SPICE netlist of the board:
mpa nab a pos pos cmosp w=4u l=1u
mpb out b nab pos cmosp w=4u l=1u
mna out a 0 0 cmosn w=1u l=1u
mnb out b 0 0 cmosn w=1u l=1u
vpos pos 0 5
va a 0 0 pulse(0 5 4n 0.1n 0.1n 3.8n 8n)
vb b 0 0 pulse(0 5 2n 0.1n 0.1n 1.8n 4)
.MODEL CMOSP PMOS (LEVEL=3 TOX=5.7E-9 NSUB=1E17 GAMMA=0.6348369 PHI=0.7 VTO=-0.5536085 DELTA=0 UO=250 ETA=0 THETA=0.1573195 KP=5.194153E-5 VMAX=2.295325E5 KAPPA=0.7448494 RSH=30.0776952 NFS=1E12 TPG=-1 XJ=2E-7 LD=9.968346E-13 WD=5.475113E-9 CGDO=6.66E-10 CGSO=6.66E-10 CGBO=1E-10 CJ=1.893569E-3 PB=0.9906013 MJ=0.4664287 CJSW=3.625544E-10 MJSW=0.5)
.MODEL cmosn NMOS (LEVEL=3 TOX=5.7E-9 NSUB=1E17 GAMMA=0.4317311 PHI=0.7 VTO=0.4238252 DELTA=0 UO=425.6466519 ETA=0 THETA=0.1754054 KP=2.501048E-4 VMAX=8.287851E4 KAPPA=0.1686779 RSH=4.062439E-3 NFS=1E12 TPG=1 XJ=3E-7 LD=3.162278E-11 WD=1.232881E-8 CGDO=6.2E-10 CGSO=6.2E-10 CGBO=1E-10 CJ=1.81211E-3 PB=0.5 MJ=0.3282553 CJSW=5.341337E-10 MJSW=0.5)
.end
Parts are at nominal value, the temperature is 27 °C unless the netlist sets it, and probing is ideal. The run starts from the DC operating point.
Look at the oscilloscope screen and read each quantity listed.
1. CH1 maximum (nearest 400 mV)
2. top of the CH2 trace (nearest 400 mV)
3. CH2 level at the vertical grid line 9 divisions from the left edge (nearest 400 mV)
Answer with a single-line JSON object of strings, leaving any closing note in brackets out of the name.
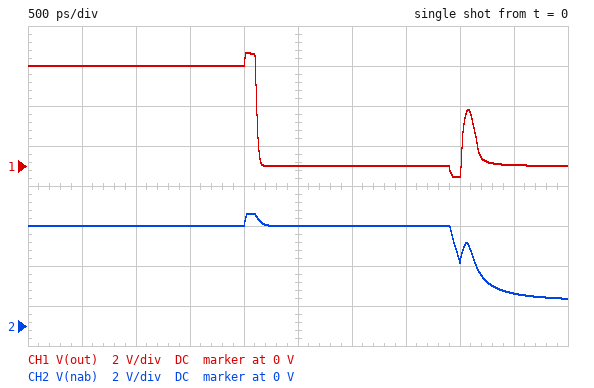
{"CH1 maximum": "5.6 V", "top of the CH2 trace": "5.6 V", "CH2 level at the vertical grid line 9 divisions from the left edge": "1.6 V"}
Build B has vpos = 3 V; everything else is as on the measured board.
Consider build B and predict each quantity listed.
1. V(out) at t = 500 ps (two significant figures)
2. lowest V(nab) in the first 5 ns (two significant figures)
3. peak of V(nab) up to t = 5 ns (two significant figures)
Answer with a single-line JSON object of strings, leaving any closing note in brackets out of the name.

{"V(out) at t = 500 ps": "3.0 V", "lowest V(nab) in the first 5 ns": "1.1 V", "peak of V(nab) up to t = 5 ns": "3.6 V"}
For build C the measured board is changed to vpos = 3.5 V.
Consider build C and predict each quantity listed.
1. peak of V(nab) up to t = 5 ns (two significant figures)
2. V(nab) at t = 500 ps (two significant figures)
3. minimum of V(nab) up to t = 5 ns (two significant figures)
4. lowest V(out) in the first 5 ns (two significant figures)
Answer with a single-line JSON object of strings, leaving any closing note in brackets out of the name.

{"peak of V(nab) up to t = 5 ns": "4.1 V", "V(nab) at t = 500 ps": "3.5 V", "minimum of V(nab) up to t = 5 ns": "1.2 V", "lowest V(out) in the first 5 ns": "-600 mV"}
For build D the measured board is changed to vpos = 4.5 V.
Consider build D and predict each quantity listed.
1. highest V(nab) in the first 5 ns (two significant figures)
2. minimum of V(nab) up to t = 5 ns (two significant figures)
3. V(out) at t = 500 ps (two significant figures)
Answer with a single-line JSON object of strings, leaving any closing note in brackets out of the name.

{"highest V(nab) in the first 5 ns": "5.1 V", "minimum of V(nab) up to t = 5 ns": "1.3 V", "V(out) at t = 500 ps": "4.5 V"}
